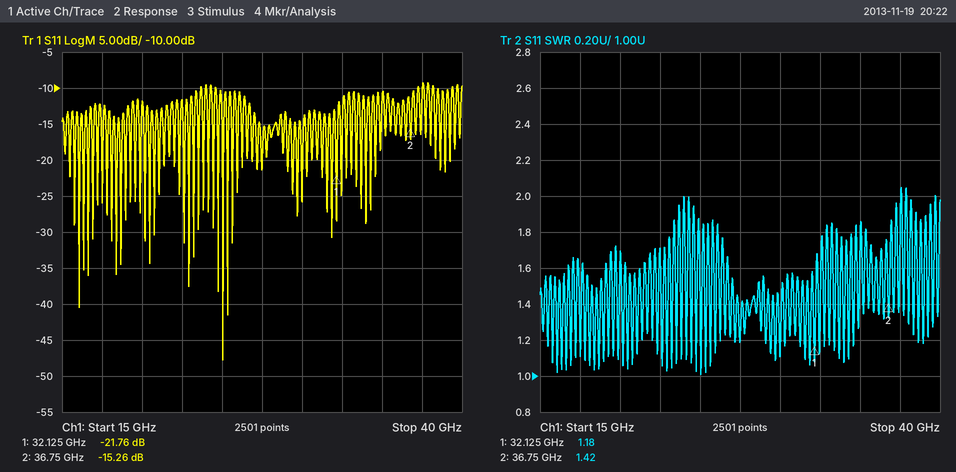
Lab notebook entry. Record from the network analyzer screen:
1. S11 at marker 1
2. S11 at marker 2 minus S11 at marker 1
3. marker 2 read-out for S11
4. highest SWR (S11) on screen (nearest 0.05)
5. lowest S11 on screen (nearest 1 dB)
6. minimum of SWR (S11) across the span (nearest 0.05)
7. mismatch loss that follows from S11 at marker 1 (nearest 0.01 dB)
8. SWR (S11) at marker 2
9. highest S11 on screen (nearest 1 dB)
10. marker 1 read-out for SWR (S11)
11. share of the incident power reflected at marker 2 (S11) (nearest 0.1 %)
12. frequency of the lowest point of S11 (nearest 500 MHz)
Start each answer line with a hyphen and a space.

- -21.76 dB
- 6.50 dB
- -15.26 dB
- 2.05
- -48 dB
- 1.00
- 0.03 dB
- 1.42
- -9 dB
- 1.18
- 3.0 %
- 25.0 GHz
